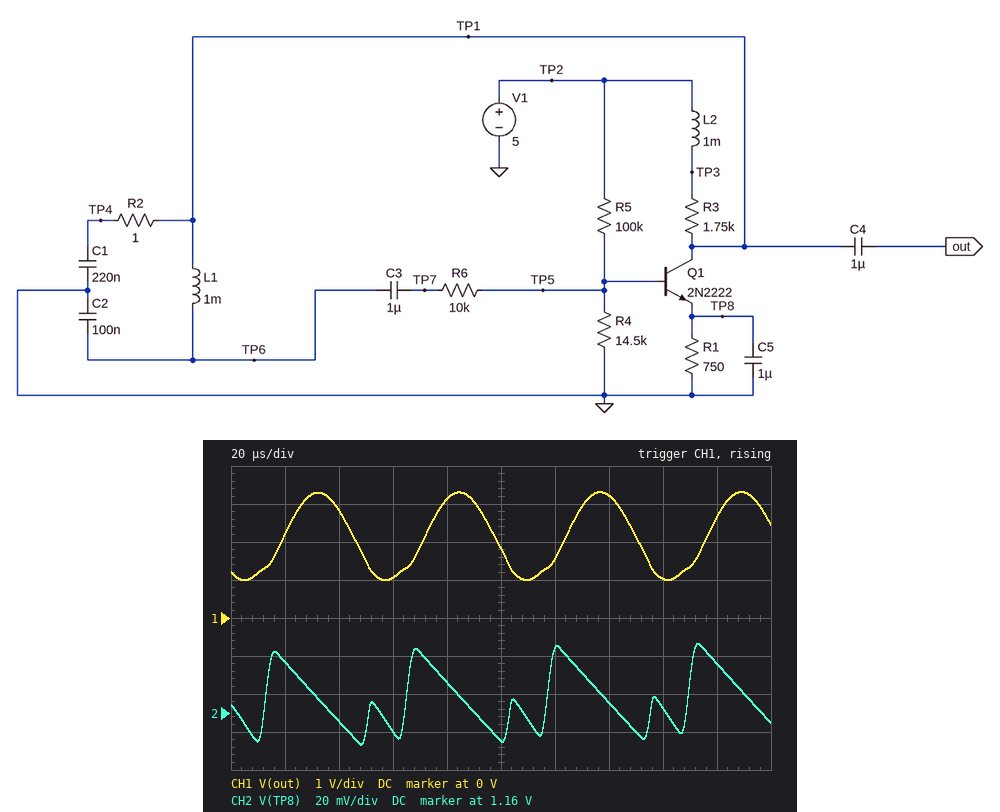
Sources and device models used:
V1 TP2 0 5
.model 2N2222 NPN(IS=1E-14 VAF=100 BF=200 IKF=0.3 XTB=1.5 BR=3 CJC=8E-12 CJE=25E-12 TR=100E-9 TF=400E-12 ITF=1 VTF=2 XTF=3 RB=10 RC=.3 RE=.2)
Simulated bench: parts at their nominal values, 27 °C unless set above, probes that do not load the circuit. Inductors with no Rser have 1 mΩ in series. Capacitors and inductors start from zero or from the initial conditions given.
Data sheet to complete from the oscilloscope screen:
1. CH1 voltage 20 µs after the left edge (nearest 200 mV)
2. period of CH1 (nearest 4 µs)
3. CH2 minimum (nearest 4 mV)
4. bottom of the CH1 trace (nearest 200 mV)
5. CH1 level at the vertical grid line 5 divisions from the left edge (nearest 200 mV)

2.2 V
52 µs
1.144 V
1.0 V
1.8 V
